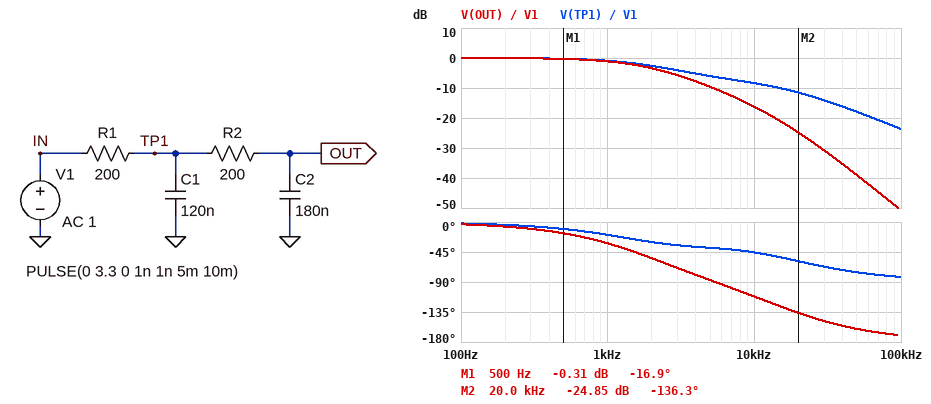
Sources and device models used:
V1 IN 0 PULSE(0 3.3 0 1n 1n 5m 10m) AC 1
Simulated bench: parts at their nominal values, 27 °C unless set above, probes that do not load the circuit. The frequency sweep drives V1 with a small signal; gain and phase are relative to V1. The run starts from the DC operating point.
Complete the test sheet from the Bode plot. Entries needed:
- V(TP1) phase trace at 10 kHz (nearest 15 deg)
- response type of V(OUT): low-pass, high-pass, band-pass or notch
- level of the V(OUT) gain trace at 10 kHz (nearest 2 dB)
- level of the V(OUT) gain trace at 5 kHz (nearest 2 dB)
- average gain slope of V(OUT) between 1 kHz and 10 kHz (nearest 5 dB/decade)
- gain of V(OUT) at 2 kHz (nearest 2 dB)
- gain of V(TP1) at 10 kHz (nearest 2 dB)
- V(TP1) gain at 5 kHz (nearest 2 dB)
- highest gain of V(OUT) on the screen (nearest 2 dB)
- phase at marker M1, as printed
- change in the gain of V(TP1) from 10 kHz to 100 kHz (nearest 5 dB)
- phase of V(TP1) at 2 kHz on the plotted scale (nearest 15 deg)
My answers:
-45 deg
low-pass
-16 dB
-10 dB
-15 dB/decade
-4 dB
-8 dB
-6 dB
0 dB
-16.9 deg
-15 dB
-30 deg
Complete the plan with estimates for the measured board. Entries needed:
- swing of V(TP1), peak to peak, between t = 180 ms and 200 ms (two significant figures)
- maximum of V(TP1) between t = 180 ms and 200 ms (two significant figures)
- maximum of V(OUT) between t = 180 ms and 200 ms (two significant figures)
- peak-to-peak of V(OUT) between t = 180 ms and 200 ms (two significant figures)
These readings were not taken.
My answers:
3.3 V
3.3 V
3.3 V
3.3 V
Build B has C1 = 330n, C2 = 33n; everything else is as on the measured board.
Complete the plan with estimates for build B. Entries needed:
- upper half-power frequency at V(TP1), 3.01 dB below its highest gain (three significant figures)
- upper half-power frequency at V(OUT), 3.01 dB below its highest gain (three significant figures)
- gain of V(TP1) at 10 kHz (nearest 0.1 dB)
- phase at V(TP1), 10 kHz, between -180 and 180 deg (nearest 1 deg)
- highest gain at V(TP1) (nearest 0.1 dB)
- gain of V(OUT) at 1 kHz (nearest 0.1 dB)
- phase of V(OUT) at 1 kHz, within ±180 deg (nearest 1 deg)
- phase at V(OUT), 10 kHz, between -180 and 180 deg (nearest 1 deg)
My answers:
2.18 kHz
2.16 kHz
-13.3 dB
-76 deg
0 dB
-0.8 dB
-27 deg
-98 deg
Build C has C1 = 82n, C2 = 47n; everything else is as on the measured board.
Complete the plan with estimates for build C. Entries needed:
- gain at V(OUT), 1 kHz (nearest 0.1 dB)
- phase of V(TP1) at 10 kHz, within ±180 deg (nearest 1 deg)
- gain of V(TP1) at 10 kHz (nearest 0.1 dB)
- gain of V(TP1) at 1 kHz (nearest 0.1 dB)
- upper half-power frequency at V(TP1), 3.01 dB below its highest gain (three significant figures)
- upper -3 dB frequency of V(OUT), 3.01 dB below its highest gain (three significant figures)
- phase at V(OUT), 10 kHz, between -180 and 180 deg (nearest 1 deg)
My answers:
-0.2 dB
-49 deg
-5.7 dB
-0.1 dB
5.68 kHz
5.15 kHz
-80 deg
